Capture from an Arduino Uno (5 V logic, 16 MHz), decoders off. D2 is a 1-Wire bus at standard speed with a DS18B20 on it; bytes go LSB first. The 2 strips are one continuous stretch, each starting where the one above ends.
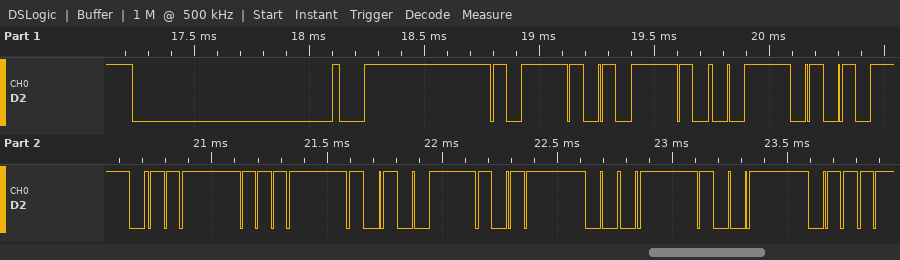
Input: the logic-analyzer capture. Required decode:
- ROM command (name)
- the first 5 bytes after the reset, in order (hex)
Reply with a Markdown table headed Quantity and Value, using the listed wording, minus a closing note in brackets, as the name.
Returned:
| Quantity | Value |
|---|---|
| ROM command | Match ROM |
| the first 5 bytes after the reset, in order | 55 28 FF D2 98 |
